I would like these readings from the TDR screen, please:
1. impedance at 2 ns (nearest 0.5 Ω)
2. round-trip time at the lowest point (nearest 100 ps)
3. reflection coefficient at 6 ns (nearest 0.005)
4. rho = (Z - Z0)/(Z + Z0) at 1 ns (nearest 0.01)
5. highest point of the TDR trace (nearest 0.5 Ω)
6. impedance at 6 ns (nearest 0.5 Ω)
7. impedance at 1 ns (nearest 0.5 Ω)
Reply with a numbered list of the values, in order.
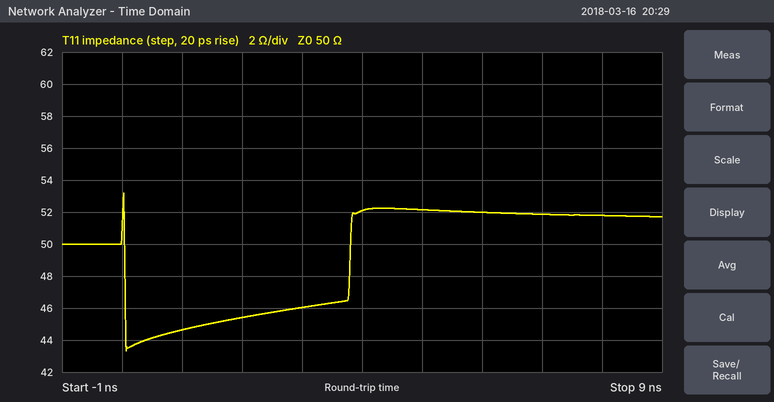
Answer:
1. 45.5 Ω
2. 100 ps
3. +0.020
4. -0.06
5. 53.0 Ω
6. 52.0 Ω
7. 44.5 Ω
